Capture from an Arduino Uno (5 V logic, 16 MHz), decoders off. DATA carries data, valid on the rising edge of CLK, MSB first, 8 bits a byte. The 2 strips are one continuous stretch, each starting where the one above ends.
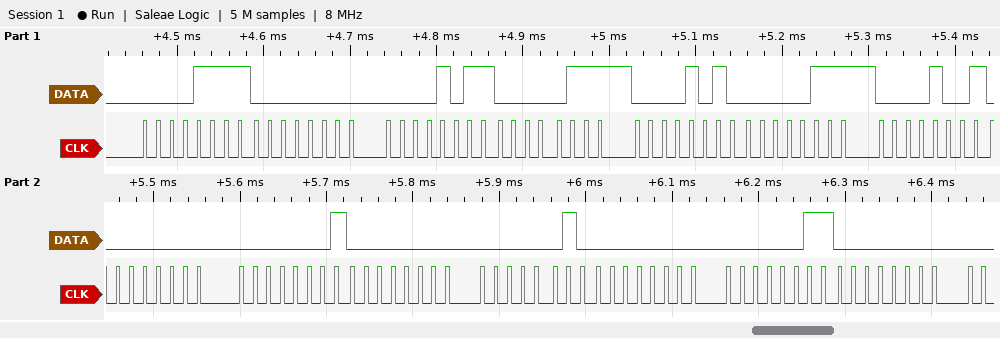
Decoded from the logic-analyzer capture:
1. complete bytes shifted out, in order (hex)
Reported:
0F 00 0B 07 0A 07 09 00 01 00 02 00 03 00
